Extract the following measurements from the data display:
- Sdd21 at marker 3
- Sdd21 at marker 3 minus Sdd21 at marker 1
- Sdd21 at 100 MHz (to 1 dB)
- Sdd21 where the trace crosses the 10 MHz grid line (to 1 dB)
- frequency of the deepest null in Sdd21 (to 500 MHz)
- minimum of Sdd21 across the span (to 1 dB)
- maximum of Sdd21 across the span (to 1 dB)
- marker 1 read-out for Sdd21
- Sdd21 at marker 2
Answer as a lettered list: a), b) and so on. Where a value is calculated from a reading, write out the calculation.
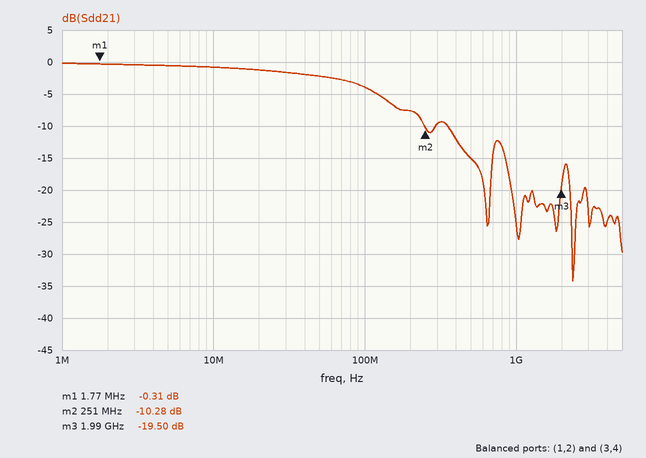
a) -19.50 dB
b) -19.5 − (-0.31) = -19.19 dB
c) -4 dB
d) -1 dB
e) 2.5 GHz
f) -34 dB
g) 0 dB
h) -0.31 dB
i) -10.28 dB
